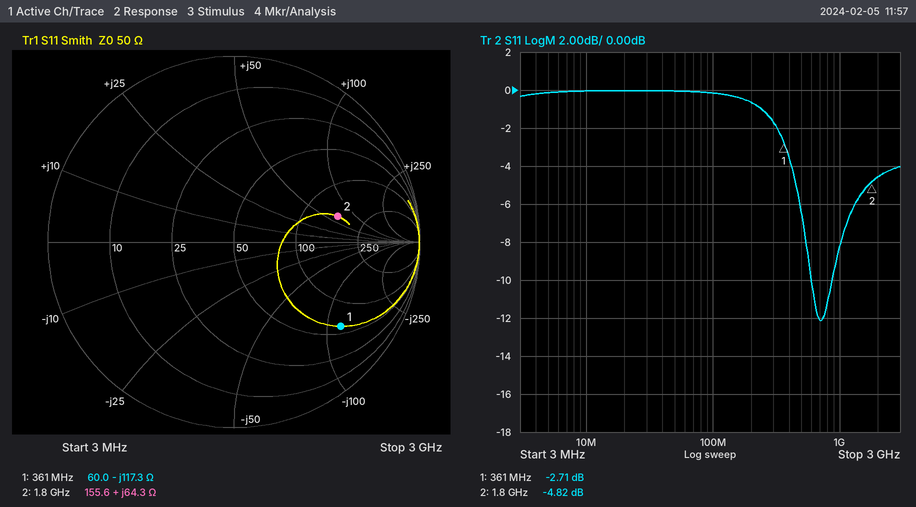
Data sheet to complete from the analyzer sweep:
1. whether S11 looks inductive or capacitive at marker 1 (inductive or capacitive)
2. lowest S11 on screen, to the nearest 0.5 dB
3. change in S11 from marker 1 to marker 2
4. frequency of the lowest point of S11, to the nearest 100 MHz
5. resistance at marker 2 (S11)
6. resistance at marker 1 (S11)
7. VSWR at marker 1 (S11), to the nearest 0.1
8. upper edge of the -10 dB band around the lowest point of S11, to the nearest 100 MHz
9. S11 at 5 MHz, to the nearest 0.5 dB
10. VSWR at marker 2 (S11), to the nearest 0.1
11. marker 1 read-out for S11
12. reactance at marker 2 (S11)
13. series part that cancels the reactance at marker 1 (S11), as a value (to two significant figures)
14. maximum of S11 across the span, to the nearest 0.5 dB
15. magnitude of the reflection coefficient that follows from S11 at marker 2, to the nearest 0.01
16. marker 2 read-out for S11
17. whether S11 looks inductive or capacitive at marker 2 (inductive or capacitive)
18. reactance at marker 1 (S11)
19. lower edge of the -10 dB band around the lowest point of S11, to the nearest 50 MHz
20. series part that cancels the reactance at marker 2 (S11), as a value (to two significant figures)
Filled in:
capacitive
-12.0 dB
-2.11 dB
700 MHz
155.6 Ω
60.0 Ω
6.5
900 MHz
0.0 dB
3.7
-2.71 dB
+64.3 Ω
52 nH
0.0 dB
0.57
-4.82 dB
inductive
-117.3 Ω
600 MHz
1.4 pF
